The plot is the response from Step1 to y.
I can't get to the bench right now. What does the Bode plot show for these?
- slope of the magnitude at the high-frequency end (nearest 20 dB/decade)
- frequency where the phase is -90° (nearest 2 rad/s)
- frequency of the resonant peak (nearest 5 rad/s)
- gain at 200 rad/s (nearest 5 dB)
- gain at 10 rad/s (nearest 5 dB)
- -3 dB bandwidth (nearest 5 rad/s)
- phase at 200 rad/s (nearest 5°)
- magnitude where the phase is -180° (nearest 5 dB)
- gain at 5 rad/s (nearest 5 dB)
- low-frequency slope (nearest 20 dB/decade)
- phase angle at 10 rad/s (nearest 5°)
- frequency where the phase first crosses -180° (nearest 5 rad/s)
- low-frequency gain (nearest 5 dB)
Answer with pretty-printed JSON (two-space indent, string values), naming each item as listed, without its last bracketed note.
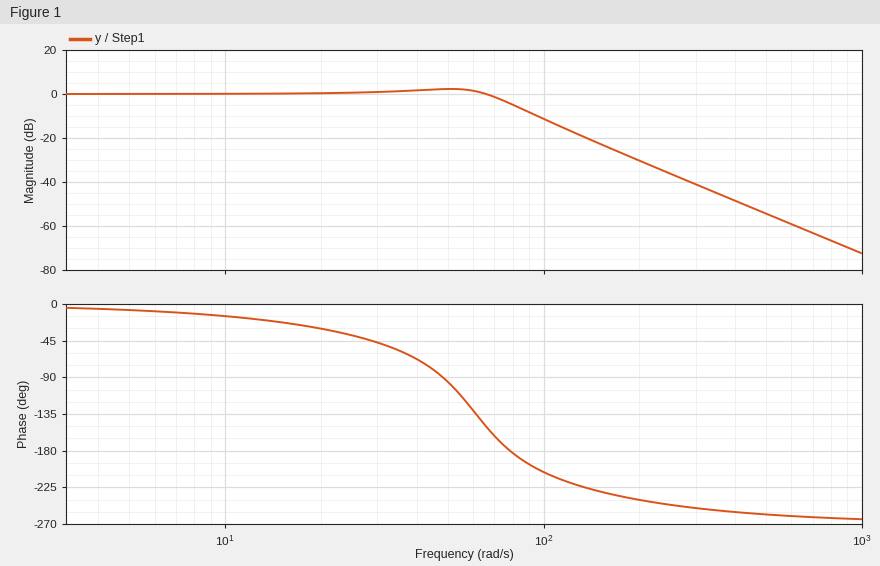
{
  "slope of the magnitude at the high-frequency end": "-60 dB/decade",
  "frequency where the phase is -90°": "48 rad/s",
  "frequency of the resonant peak": "50 rad/s",
  "gain at 200 rad/s": "-30 dB",
  "gain at 10 rad/s": "0 dB",
  "-3 dB bandwidth": "75 rad/s",
  "phase at 200 rad/s": "-240°",
  "magnitude where the phase is -180°": "-5 dB",
  "gain at 5 rad/s": "0 dB",
  "low-frequency slope": "0 dB/decade",
  "phase angle at 10 rad/s": "-15°",
  "frequency where the phase first crosses -180°": "80 rad/s",
  "low-frequency gain": "0 dB"
}
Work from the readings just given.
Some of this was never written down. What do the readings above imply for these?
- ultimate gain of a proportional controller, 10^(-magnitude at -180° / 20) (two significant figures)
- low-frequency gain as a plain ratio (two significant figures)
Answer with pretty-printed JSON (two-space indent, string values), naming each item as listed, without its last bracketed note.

{
  "ultimate gain of a proportional controller, 10^(-magnitude at -180° / 20)": "1.8",
  "low-frequency gain as a plain ratio": "1.0"
}
